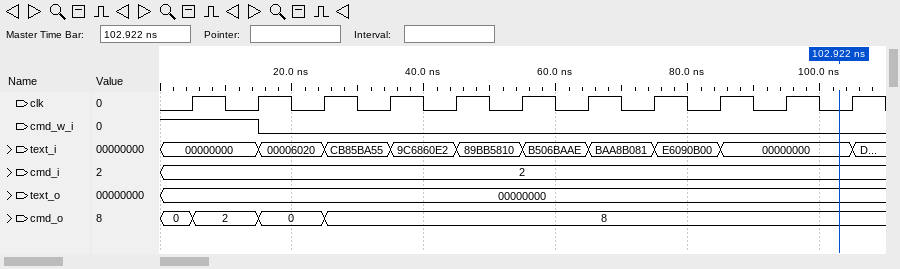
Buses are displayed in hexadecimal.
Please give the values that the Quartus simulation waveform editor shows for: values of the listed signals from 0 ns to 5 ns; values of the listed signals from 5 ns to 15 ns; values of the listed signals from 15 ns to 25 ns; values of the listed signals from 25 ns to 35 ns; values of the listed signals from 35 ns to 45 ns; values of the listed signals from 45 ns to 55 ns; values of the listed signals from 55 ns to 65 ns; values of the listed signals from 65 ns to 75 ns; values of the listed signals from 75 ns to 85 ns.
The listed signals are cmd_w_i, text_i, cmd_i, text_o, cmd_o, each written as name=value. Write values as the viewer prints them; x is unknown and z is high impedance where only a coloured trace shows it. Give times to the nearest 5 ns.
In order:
cmd_w_i=1, text_i=00000000, cmd_i=2, text_o=00000000, cmd_o=0
cmd_w_i=1, text_i=00000000, cmd_i=2, text_o=00000000, cmd_o=2
cmd_w_i=0, text_i=00006020, cmd_i=2, text_o=00000000, cmd_o=0
cmd_w_i=0, text_i=CB85BA55, cmd_i=2, text_o=00000000, cmd_o=8
cmd_w_i=0, text_i=9C6860E2, cmd_i=2, text_o=00000000, cmd_o=8
cmd_w_i=0, text_i=89BB5810, cmd_i=2, text_o=00000000, cmd_o=8
cmd_w_i=0, text_i=B506BAAE, cmd_i=2, text_o=00000000, cmd_o=8
cmd_w_i=0, text_i=BAA8B081, cmd_i=2, text_o=00000000, cmd_o=8
cmd_w_i=0, text_i=E6090B00, cmd_i=2, text_o=00000000, cmd_o=8
